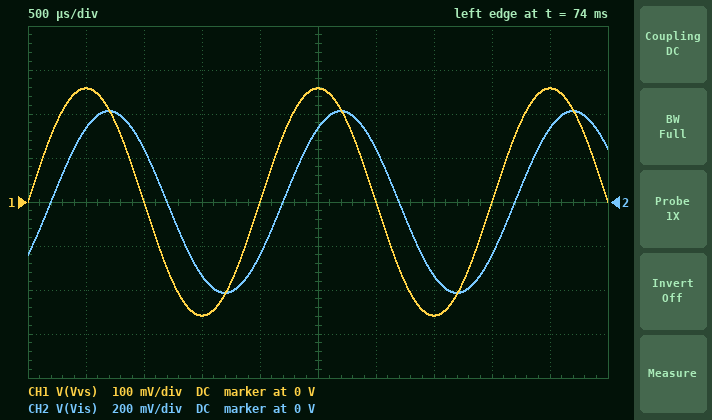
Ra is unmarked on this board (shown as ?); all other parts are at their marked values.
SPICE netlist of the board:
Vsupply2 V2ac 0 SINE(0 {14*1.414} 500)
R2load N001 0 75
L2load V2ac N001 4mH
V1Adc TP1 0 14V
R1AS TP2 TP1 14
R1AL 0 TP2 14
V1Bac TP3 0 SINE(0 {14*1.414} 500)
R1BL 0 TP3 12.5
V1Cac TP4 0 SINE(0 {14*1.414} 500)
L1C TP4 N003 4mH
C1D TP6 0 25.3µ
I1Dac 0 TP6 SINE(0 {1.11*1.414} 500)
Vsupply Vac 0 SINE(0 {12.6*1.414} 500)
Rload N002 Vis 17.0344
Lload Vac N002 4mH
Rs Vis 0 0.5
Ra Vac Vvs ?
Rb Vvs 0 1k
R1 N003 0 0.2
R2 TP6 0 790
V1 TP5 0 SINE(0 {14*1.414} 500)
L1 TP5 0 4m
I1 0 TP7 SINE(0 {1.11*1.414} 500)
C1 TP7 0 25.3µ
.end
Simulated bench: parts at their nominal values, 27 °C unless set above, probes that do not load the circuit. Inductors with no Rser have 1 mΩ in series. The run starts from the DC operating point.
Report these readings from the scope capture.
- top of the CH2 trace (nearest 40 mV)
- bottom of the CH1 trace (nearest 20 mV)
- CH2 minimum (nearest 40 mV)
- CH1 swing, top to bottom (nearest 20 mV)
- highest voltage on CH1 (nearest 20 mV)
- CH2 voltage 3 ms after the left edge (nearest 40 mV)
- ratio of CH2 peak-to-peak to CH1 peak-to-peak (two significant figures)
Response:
400 mV
-260 mV
-400 mV
520 mV
260 mV
240 mV
1.6
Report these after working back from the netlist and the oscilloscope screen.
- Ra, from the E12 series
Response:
68 kΩ
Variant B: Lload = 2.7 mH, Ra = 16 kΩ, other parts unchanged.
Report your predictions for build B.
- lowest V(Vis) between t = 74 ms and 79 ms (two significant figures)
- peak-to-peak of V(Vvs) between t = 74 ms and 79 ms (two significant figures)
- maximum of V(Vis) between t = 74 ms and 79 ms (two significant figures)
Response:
-460 mV
2.1 V
460 mV
